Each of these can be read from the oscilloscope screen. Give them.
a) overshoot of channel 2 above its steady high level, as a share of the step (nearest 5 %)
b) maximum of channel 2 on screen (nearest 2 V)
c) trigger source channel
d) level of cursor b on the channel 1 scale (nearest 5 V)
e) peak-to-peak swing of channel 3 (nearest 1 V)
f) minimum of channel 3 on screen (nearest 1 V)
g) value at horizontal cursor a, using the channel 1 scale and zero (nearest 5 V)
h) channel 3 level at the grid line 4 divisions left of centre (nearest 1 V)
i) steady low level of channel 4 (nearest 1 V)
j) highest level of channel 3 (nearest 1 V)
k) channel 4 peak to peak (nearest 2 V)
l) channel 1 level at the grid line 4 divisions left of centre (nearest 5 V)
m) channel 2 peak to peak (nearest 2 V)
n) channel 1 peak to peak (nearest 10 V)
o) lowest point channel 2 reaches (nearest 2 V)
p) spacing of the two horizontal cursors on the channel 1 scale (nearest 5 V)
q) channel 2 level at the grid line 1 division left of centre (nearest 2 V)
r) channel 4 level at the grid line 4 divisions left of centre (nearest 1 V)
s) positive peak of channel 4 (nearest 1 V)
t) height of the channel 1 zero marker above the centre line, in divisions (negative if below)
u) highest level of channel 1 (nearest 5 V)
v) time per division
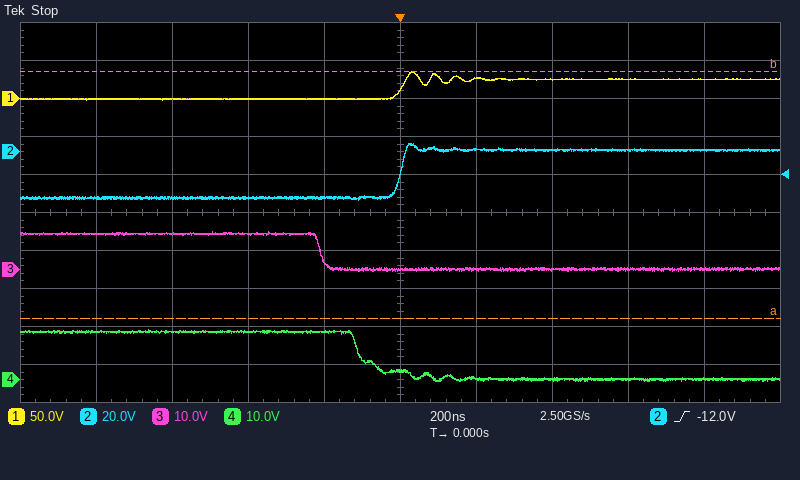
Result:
15 %
4 V
channel 2
35 V
11 V
-1 V
-290 V
9 V
0 V
10 V
14 V
0 V
30 V
40 V
-26 V
325 V
-24 V
13 V
13 V
+3.0 div
35 V
200 ns
